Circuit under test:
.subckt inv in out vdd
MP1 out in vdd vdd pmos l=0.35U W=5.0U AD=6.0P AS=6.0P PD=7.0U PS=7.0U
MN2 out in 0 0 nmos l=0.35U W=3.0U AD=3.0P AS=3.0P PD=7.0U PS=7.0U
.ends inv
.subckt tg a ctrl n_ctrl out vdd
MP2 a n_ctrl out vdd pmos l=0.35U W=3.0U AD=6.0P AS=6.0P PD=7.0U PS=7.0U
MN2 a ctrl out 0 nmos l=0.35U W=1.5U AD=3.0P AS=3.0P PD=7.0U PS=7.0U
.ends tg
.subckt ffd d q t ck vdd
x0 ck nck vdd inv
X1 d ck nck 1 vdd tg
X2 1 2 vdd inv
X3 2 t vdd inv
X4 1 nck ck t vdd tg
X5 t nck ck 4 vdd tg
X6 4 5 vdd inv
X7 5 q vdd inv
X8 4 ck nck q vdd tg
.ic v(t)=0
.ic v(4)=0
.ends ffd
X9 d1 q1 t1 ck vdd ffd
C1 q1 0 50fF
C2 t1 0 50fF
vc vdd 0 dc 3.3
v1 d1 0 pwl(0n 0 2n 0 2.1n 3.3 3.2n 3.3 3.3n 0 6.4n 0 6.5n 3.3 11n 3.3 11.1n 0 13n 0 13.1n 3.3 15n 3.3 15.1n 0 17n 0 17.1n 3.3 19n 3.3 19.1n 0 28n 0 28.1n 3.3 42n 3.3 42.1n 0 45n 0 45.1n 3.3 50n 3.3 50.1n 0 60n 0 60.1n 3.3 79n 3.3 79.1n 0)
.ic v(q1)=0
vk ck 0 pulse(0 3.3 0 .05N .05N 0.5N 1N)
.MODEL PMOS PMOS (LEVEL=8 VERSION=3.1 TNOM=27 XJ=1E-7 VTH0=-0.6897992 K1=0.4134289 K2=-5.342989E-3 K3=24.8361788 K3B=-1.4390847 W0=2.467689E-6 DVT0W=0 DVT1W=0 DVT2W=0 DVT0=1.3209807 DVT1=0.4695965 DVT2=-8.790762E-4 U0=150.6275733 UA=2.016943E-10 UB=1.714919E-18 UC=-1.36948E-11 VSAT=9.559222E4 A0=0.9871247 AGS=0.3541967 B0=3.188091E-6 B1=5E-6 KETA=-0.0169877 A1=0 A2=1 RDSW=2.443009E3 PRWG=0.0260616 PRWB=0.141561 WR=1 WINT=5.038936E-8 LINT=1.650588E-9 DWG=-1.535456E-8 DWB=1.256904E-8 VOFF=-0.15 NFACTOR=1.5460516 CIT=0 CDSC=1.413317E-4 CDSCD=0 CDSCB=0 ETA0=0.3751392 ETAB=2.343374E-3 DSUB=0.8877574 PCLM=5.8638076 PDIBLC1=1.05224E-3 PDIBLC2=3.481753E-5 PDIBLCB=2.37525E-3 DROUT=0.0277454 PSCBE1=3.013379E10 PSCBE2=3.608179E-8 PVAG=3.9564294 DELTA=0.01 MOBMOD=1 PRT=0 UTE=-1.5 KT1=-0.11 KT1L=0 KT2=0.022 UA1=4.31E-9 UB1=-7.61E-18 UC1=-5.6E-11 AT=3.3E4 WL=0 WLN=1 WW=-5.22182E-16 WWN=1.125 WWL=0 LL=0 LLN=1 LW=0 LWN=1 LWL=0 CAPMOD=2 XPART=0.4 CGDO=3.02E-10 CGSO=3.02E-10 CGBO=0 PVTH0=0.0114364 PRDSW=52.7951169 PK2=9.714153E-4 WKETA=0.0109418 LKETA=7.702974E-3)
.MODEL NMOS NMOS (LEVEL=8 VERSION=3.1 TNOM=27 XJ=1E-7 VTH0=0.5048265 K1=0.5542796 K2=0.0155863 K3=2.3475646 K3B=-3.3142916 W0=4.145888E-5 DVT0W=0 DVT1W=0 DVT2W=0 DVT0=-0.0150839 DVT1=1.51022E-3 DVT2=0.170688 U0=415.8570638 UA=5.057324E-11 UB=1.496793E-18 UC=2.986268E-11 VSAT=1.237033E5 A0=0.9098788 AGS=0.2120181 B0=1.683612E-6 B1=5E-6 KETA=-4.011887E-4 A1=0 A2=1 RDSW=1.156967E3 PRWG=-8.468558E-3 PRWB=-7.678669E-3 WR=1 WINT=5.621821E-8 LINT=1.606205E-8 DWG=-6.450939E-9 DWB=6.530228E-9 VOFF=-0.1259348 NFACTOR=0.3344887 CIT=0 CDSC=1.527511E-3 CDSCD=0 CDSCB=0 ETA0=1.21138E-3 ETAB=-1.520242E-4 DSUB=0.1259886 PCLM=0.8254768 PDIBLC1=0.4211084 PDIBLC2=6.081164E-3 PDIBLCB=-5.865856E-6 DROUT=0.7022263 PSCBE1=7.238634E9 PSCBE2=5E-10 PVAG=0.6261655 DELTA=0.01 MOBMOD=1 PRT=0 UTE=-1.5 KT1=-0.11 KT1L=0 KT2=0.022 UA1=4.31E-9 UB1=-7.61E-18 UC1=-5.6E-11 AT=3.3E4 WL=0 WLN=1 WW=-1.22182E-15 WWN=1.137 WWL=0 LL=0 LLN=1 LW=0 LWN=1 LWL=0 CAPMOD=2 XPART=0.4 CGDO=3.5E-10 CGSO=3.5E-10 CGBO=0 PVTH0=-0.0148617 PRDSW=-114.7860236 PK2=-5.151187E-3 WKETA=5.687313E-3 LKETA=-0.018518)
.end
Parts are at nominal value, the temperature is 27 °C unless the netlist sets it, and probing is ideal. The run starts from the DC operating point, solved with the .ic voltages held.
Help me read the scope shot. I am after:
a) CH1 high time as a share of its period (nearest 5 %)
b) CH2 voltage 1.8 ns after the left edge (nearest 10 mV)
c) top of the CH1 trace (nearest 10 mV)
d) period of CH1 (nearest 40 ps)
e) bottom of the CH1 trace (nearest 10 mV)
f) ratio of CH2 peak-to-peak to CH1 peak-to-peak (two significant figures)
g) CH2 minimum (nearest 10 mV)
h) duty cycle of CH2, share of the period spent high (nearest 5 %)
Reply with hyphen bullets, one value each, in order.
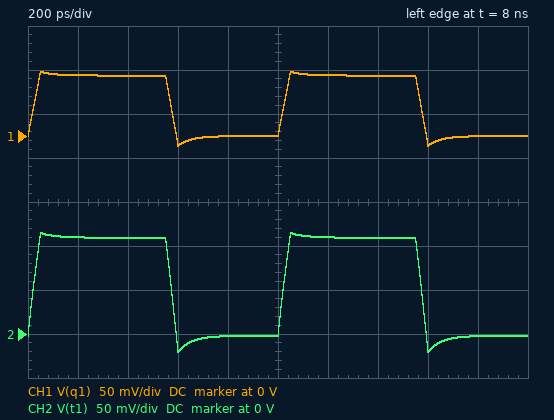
- 55 %
- 0 V
- 70 mV
- 1.00 ns
- -10 mV
- 1.6
- -20 mV
- 55 %
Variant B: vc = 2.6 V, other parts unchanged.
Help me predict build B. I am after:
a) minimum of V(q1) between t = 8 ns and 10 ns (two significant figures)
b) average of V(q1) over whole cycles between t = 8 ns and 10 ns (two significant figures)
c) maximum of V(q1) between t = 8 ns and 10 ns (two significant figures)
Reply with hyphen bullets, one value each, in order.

- -7.5 mV
- 37 mV
- 72 mV
